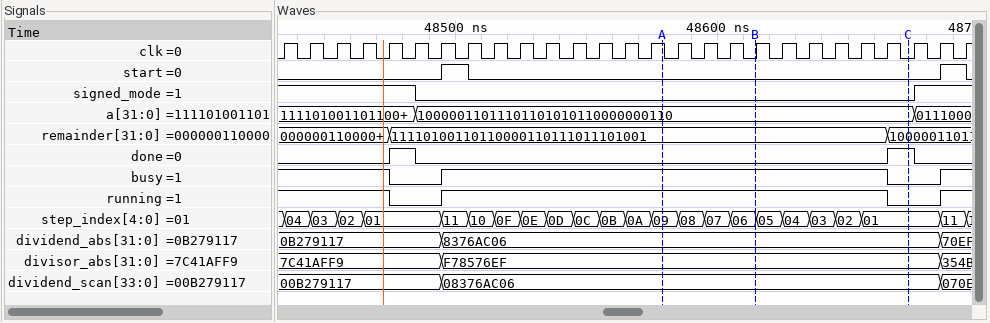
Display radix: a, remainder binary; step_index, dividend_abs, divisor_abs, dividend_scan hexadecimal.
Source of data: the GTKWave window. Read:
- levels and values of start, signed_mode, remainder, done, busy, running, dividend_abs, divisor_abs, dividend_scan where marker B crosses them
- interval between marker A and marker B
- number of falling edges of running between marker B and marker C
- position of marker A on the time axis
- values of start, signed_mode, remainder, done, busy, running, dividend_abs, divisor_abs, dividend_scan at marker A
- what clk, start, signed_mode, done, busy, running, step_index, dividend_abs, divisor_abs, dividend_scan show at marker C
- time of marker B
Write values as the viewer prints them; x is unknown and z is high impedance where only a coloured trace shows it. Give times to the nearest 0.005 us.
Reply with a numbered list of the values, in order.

1. start=0, signed_mode=0, remainder=11110100110110000110111011101001, done=0, busy=1, running=1, dividend_abs=8376AC06, divisor_abs=F78576EF, dividend_scan=08376AC06
2. 0.035 us
3. 1
4. 48.58 us
5. start=0, signed_mode=0, remainder=11110100110110000110111011101001, done=0, busy=1, running=1, dividend_abs=8376AC06, divisor_abs=F78576EF, dividend_scan=08376AC06
6. clk=0, start=0, signed_mode=0, done=1, busy=0, running=0, step_index=01, dividend_abs=8376AC06, divisor_abs=F78576EF, dividend_scan=08376AC06
7. 48.615 us
